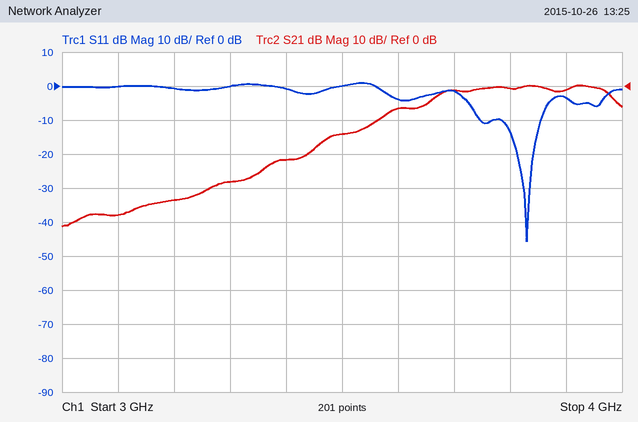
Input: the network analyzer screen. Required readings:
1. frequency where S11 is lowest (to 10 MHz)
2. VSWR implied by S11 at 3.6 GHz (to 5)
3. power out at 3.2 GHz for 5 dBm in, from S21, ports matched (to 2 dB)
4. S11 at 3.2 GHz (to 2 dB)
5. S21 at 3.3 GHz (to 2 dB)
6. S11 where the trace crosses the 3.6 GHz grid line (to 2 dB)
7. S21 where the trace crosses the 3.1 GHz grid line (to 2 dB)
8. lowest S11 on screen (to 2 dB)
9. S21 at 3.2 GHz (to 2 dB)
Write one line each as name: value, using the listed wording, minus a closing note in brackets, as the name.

frequency where S11 is lowest: 3.83 GHz
VSWR implied by S11 at 3.6 GHz: 5
power out at 3.2 GHz for 5 dBm in, from S21, ports matched: -28 dBm
S11 at 3.2 GHz: 0 dB
S21 at 3.3 GHz: -28 dB
S11 where the trace crosses the 3.6 GHz grid line: -4 dB
S21 where the trace crosses the 3.1 GHz grid line: -38 dB
lowest S11 on screen: -46 dB
S21 at 3.2 GHz: -34 dB
